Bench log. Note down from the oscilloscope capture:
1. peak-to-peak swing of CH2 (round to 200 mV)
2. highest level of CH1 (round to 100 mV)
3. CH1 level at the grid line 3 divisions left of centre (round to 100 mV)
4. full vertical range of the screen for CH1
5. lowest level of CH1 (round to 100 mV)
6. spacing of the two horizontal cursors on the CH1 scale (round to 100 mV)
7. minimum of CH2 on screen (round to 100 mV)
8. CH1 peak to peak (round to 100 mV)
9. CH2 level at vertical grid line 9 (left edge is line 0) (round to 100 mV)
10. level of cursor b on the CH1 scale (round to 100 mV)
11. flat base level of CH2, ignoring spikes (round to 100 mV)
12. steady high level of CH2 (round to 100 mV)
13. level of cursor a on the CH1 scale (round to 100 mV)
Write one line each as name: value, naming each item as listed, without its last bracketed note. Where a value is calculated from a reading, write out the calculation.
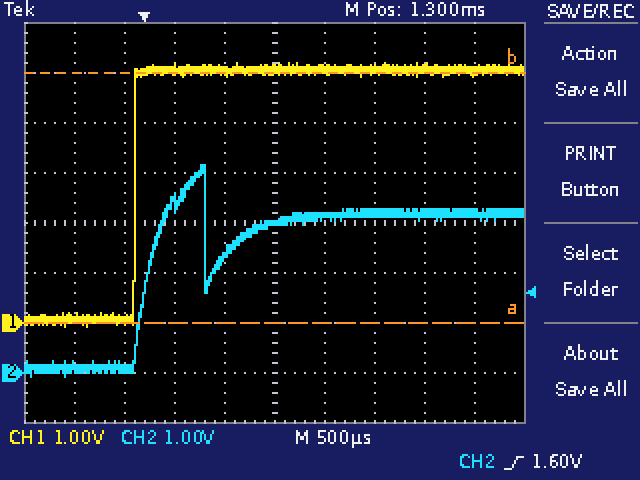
peak-to-peak swing of CH2: 4.2 V
highest level of CH1: 5.2 V
CH1 level at the grid line 3 divisions left of centre: 100 mV
full vertical range of the screen for CH1: 8 V
lowest level of CH1: -100 mV
spacing of the two horizontal cursors on the CH1 scale: 5.0 V
minimum of CH2 on screen: -100 mV
CH1 peak to peak: 5.2 V − (-100 mV) = 5.3 V
CH2 level at vertical grid line 9 (left edge is line 0): 3.2 V
level of cursor b on the CH1 scale: 5.0 V
flat base level of CH2, ignoring spikes: 100 mV
steady high level of CH2: 3.2 V
level of cursor a on the CH1 scale: 0.0 V
